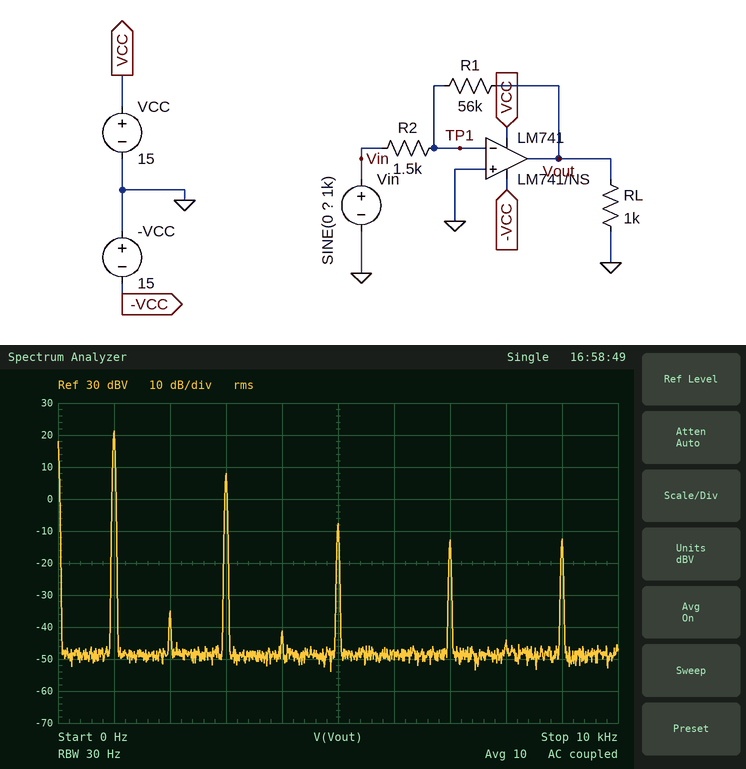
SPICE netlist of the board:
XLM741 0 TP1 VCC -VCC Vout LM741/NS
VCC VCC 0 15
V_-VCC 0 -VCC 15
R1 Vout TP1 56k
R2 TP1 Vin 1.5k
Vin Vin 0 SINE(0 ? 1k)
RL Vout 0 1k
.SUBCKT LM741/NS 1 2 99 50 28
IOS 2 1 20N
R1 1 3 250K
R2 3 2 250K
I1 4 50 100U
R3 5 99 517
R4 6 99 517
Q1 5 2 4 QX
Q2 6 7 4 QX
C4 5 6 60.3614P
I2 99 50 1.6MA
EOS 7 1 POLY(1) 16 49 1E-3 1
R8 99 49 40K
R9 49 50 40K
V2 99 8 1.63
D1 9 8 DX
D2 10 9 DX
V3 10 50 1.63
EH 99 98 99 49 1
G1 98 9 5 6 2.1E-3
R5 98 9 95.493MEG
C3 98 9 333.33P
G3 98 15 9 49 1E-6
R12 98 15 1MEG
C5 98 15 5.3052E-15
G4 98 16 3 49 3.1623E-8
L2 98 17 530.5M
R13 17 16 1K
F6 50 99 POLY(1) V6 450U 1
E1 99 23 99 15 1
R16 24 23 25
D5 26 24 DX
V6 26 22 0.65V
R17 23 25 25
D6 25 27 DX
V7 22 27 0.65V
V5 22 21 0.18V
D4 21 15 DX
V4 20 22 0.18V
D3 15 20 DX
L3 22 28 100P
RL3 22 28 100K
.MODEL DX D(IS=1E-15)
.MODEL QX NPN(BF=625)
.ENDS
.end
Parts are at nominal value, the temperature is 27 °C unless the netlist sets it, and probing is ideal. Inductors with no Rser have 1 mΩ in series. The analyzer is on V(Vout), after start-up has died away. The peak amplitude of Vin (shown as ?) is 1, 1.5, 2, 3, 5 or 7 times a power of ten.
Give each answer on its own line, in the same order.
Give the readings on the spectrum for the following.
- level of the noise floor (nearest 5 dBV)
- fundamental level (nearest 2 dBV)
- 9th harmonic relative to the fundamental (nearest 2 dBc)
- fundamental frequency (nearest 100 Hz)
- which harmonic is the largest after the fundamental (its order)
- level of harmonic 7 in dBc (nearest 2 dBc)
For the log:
-50 dBV
22 dBV
-34 dBc
1.0 kHz
3
-34 dBc
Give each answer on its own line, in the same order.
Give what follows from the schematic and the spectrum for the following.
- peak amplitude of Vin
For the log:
700 mV
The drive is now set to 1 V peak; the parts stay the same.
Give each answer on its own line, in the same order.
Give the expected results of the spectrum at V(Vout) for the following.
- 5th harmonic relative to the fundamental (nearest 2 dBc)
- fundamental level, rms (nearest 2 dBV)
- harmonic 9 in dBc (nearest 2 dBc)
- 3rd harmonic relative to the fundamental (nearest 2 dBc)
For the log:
-20 dBc
22 dBV
-44 dBc
-12 dBc
